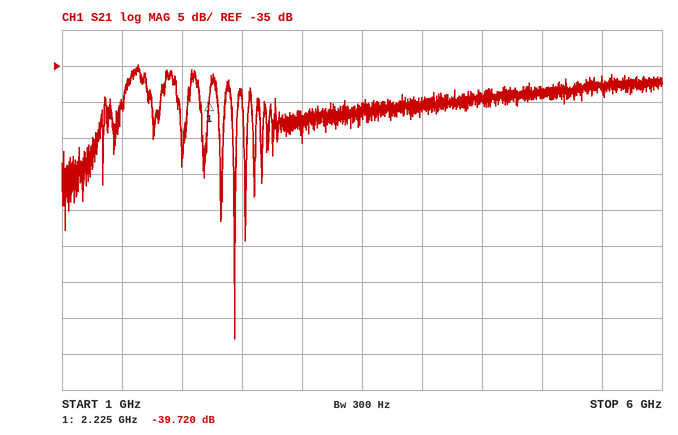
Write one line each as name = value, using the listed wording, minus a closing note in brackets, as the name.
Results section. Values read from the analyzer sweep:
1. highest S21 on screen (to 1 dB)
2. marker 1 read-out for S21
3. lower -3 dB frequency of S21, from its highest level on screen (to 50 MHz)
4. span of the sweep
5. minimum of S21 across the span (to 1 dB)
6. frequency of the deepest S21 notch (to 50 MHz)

highest S21 on screen = -35 dB
marker 1 read-out for S21 = -39.720 dB
lower -3 dB frequency of S21, from its highest level on screen = 1.55 GHz
span of the sweep = 5 GHz
minimum of S21 across the span = -73 dB
frequency of the deepest S21 notch = 2.45 GHz
